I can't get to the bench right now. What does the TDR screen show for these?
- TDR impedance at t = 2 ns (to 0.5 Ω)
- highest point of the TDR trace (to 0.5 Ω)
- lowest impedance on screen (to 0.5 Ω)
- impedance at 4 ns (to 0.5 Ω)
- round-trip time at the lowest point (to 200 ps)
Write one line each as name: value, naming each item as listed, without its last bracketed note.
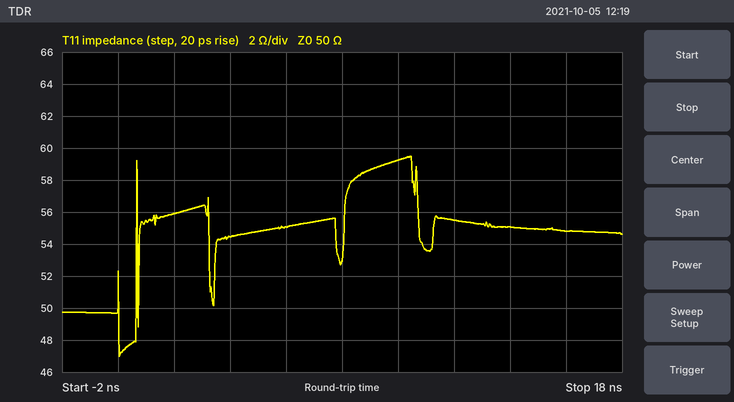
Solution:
TDR impedance at t = 2 ns: 56.0 Ω
highest point of the TDR trace: 59.5 Ω
lowest impedance on screen: 47.0 Ω
impedance at 4 ns: 54.5 Ω
round-trip time at the lowest point: 0.0 ns
